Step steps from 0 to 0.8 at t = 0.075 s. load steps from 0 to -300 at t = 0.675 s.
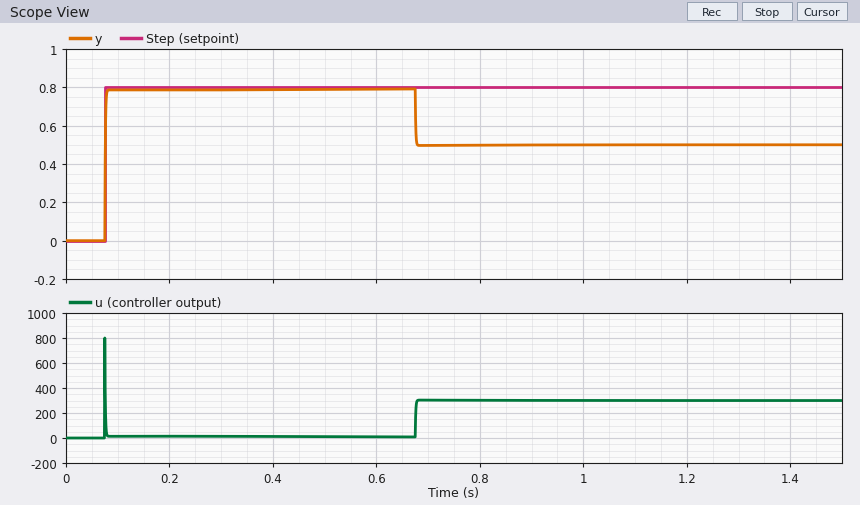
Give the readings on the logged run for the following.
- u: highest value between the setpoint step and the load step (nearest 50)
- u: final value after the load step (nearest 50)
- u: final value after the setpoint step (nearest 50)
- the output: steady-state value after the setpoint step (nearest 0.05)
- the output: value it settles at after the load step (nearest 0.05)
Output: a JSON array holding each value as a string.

["800", "300", "0", "0.80", "0.50"]
